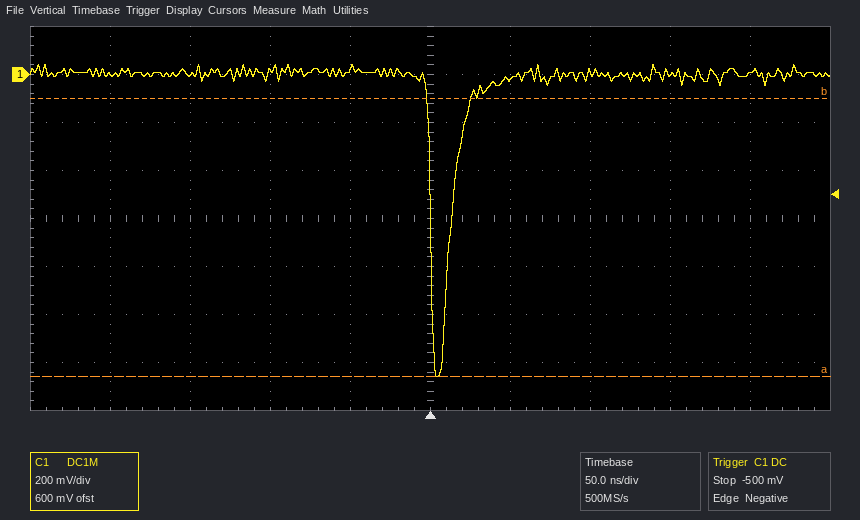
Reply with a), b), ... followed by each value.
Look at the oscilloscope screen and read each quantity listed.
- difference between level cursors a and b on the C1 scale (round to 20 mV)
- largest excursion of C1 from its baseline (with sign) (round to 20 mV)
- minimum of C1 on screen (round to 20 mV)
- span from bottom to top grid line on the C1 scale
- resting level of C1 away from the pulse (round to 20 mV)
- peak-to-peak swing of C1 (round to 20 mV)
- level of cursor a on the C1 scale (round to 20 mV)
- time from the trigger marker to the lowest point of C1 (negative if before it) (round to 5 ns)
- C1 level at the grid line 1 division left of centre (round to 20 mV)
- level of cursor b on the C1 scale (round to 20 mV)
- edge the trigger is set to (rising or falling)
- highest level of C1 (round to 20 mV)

a) 1.16 V
b) -1.26 V
c) -1.26 V
d) 1.6 V
e) 0 mV
f) 1.30 V
g) -1.26 V
h) +5 ns
i) 20 mV
j) -100 mV
k) falling
l) 40 mV
